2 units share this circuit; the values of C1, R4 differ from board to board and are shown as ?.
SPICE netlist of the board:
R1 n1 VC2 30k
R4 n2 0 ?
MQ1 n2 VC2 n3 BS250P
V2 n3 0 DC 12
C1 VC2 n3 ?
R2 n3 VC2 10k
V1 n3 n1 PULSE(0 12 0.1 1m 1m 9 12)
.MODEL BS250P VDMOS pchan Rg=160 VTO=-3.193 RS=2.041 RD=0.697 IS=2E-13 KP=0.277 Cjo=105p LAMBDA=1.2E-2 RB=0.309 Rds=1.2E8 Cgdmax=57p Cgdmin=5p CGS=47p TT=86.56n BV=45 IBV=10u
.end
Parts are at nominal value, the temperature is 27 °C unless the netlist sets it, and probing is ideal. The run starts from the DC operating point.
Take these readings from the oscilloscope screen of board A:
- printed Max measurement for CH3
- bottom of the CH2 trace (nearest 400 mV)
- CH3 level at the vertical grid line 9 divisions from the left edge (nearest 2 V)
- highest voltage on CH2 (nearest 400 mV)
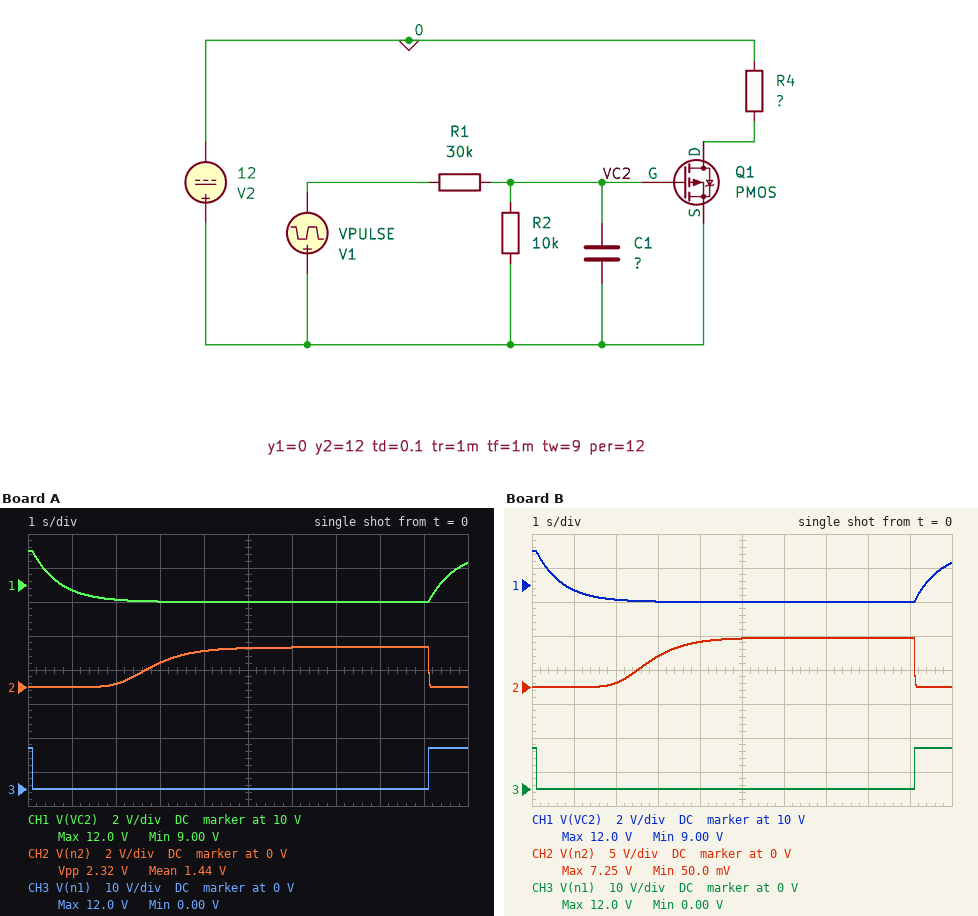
12.0 V
0 V
0 V
2.4 V
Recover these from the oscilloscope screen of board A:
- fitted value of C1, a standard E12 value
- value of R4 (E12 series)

82 µF
82 kΩ
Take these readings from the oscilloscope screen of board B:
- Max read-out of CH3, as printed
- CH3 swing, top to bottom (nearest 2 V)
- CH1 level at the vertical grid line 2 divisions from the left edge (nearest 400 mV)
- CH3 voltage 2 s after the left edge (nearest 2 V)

12.0 V
12 V
9.2 V
0 V
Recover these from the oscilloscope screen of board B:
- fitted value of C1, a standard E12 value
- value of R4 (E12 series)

82 µF
270 kΩ
